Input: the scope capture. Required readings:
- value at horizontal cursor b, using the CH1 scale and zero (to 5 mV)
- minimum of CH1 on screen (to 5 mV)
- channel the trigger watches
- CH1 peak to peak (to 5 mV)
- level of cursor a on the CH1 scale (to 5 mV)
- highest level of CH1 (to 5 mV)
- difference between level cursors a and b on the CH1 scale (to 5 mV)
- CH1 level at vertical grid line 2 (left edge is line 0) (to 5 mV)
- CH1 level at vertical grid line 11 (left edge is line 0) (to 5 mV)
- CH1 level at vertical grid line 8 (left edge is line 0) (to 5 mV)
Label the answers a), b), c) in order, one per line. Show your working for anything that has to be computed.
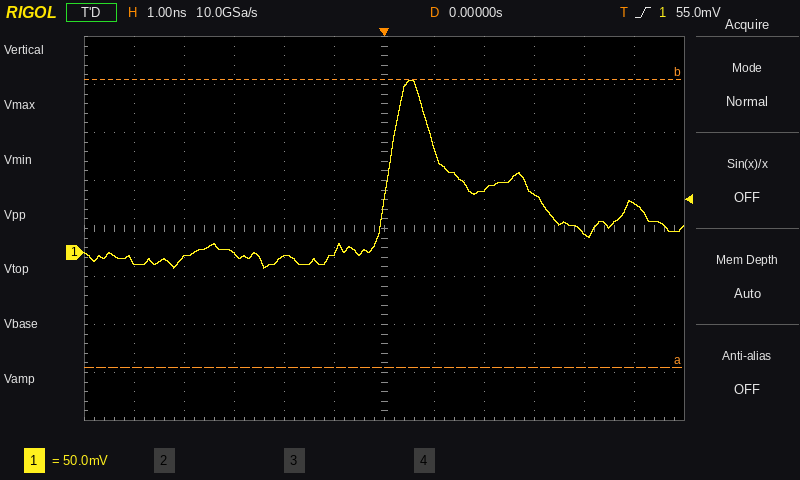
a) 180 mV
b) -15 mV
c) CH1
d) 180 mV − (-15 mV) = 195 mV
e) -120 mV
f) 180 mV
g) 300 mV
h) -5 mV
i) 50 mV
j) 65 mV
